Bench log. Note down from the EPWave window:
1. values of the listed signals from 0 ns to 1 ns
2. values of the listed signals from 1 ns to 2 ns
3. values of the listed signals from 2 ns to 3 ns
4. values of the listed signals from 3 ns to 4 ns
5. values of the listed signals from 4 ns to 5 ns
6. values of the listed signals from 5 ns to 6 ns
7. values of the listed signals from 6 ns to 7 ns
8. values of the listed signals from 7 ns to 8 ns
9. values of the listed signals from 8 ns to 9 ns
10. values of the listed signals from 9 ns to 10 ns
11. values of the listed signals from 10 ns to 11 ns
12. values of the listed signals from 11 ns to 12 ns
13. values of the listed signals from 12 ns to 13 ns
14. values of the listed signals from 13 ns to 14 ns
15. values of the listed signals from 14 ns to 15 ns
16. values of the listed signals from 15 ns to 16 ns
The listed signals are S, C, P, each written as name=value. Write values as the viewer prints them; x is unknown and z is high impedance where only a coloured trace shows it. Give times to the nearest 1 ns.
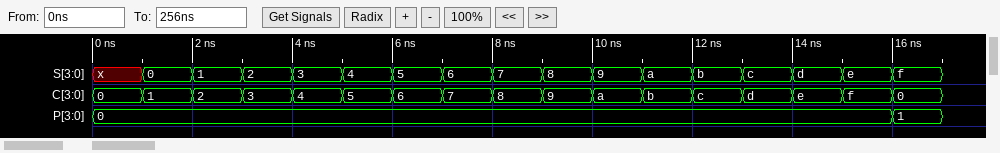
S=x, C=0, P=0
S=0, C=1, P=0
S=1, C=2, P=0
S=2, C=3, P=0
S=3, C=4, P=0
S=4, C=5, P=0
S=5, C=6, P=0
S=6, C=7, P=0
S=7, C=8, P=0
S=8, C=9, P=0
S=9, C=a, P=0
S=a, C=b, P=0
S=b, C=c, P=0
S=c, C=d, P=0
S=d, C=e, P=0
S=e, C=f, P=0
